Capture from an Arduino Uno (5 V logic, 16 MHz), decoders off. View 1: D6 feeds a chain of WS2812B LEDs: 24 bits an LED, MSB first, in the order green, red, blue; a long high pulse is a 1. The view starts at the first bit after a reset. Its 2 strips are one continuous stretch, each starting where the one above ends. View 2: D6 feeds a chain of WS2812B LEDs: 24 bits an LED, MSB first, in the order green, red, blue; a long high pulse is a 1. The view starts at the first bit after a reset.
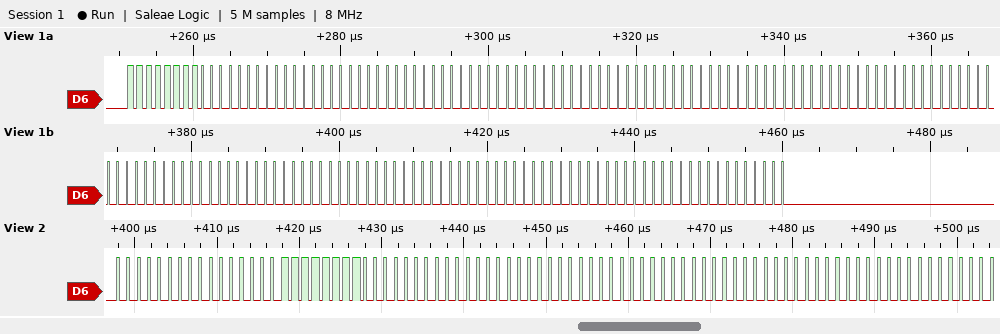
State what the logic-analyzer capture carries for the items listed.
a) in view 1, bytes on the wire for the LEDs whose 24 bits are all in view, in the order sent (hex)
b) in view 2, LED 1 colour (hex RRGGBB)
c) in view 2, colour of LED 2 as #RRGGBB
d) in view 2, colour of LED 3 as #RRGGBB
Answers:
FF 00 00 00 00 00 00 00 00 00 00 00 00 00 00 00 00 00 00 00 00
#0000FF
#000000
#000000
